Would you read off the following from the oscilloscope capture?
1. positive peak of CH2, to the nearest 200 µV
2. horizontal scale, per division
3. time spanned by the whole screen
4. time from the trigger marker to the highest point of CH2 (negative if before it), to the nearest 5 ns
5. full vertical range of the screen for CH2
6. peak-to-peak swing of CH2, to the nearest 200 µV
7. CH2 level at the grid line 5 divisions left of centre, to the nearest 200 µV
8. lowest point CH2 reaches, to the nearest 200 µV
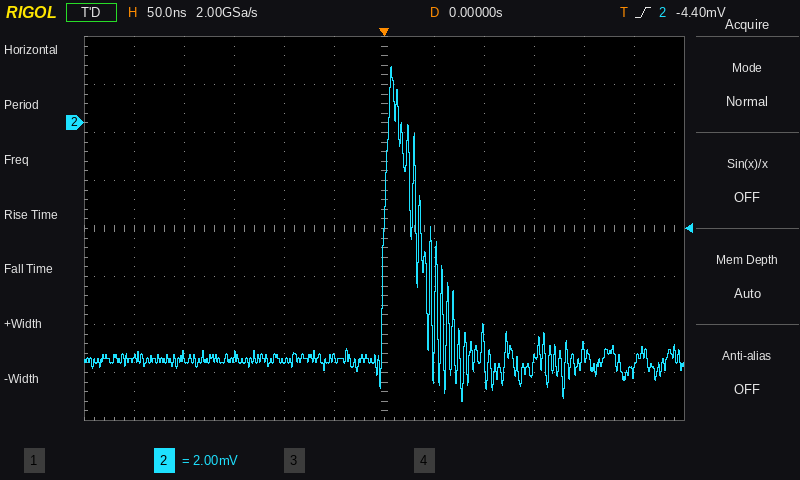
2.4 mV
50 ns
600 ns
+5 ns
16 mV
14.0 mV
-9.8 mV
-11.6 mV
